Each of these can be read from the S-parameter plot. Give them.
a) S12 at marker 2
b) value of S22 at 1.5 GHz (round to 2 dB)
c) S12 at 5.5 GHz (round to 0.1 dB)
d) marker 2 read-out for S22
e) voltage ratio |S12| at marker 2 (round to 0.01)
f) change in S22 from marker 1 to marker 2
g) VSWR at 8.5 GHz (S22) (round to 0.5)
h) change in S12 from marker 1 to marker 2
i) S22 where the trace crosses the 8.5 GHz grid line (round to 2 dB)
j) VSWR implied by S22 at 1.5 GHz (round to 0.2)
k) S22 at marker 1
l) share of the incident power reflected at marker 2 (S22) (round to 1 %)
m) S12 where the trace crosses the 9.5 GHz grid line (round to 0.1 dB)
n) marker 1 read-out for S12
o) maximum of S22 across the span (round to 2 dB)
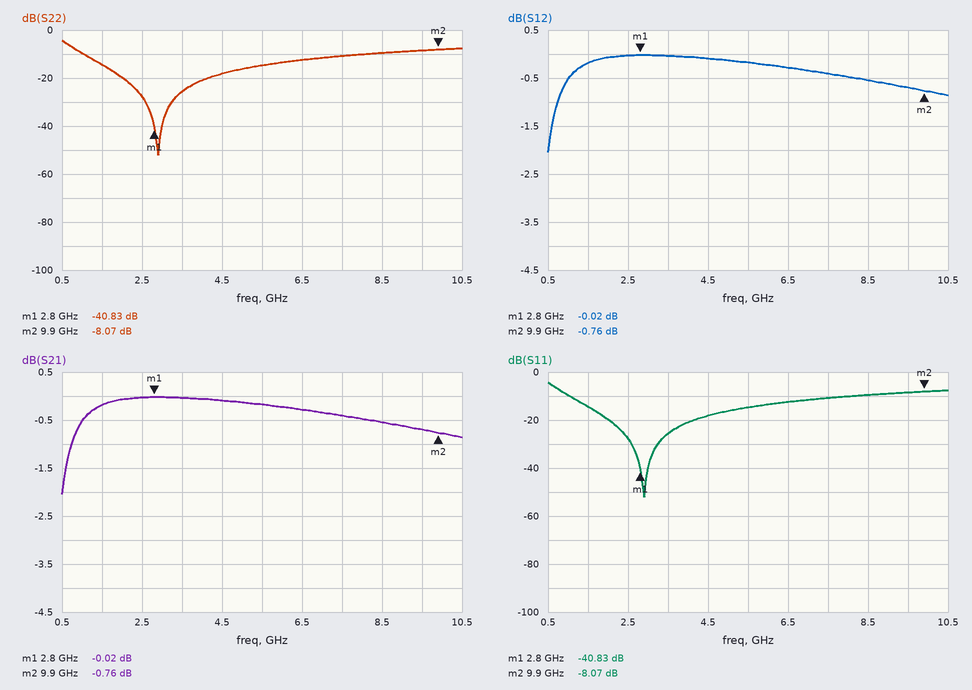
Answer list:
-0.76 dB
-14 dB
-0.2 dB
-8.07 dB
0.92
32.76 dB
2.0
-0.74 dB
-10 dB
1.4
-40.83 dB
16 %
-0.7 dB
-0.02 dB
-4 dB
